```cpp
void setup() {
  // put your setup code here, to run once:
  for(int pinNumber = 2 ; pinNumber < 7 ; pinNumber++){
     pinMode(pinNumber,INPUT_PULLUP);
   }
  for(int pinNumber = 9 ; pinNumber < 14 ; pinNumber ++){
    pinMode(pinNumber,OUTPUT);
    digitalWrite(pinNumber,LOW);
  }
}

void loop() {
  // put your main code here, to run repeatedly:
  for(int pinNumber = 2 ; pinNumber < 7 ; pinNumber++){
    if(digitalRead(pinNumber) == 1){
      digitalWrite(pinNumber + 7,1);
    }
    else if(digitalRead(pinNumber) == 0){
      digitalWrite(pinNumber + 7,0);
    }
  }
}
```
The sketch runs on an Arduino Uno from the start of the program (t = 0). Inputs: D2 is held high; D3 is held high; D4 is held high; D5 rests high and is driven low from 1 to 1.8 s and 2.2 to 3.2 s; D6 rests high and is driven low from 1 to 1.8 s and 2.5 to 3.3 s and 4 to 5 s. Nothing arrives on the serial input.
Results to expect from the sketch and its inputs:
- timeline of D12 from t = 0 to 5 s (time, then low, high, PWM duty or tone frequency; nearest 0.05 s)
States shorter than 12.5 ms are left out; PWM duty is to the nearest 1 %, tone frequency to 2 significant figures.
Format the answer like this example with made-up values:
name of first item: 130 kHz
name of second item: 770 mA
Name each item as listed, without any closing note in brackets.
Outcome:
timeline of D12 from t = 0 to 5 s: 0 s high; 1 s low; 1.8 s high; 2.2 s low; 3.2 s high
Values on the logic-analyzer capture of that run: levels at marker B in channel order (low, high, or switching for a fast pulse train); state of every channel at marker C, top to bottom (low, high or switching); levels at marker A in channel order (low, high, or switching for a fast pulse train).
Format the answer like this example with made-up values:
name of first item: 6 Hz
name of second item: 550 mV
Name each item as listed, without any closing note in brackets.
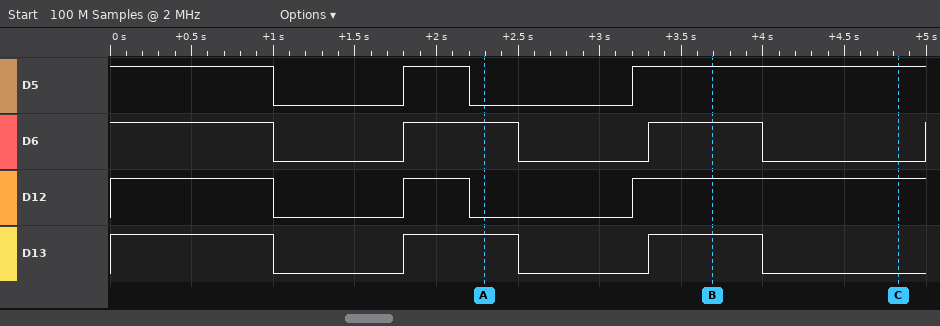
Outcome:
levels at marker B in channel order: D5 high, D6 high, D12 high, D13 high
state of every channel at marker C, top to bottom: D5 high, D6 low, D12 high, D13 low
levels at marker A in channel order: D5 low, D6 high, D12 low, D13 high
